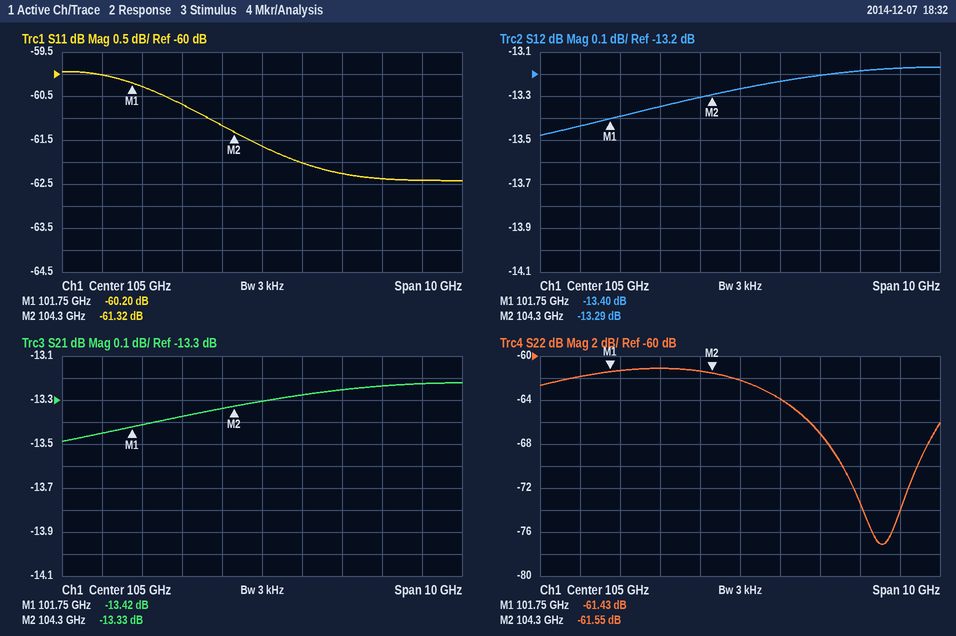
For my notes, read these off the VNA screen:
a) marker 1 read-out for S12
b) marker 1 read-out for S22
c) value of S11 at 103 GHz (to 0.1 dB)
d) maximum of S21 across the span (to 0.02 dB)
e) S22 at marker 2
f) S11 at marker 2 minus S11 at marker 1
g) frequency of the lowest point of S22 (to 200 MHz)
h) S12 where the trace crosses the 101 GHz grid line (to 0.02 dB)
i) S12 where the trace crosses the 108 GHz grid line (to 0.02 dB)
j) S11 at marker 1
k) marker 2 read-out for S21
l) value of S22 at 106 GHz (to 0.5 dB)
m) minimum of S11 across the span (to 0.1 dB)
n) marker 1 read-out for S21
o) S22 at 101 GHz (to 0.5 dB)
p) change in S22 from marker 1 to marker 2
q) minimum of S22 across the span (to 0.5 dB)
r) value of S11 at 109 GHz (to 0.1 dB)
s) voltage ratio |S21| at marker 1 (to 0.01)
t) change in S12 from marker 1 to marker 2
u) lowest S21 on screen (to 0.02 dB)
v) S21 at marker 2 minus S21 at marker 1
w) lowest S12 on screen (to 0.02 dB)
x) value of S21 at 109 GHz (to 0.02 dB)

-13.40 dB
-61.43 dB
-60.7 dB
-13.22 dB
-61.55 dB
-1.12 dB
108.6 GHz
-13.44 dB
-13.18 dB
-60.20 dB
-13.33 dB
-64.0 dB
-62.4 dB
-13.42 dB
-62.0 dB
-0.12 dB
-77.0 dB
-62.4 dB
0.21
0.11 dB
-13.48 dB
0.09 dB
-13.48 dB
-13.22 dB
